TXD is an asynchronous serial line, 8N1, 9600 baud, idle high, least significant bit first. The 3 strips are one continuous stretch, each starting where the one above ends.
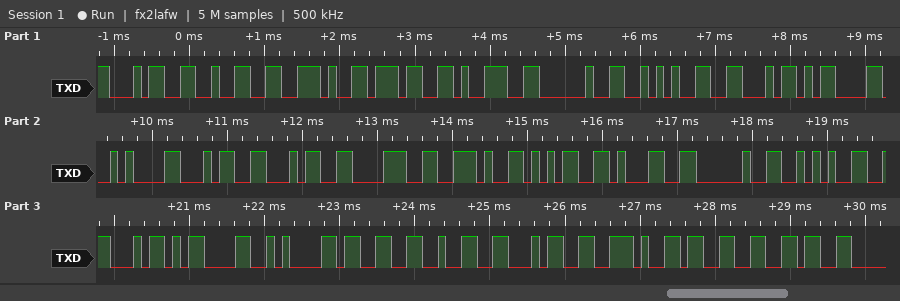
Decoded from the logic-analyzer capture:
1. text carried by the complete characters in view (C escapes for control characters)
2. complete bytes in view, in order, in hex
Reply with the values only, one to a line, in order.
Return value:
"42.79 *F\r\n448.51 *F\r\n324.36"
34 32 2E 37 39 20 2A 46 0D 0A 34 34 38 2E 35 31 20 2A 46 0D 0A 33 32 34 2E 33 36
